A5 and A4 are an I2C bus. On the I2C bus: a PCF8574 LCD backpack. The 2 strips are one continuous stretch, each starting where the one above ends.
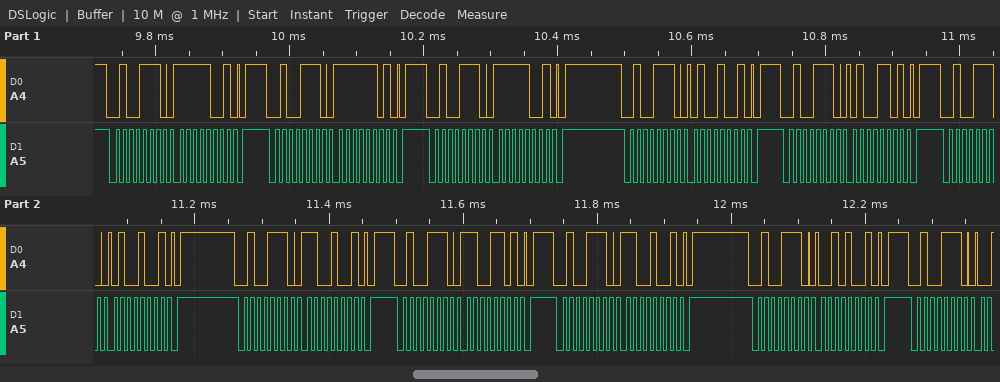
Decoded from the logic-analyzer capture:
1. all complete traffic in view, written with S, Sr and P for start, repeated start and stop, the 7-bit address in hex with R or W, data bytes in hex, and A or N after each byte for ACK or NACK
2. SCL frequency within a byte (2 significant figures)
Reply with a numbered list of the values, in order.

1. S 27W A F9 A P S 27W A FD A P S 27W A F9 A P S 27W A 49 A P S 27W A 4D A P S 27W A 49 A P S 27W A C9 A P S 27W A CD A P S 27W A C9 A P S 27W A 29 A P S 27W A
2. 100 kHz
